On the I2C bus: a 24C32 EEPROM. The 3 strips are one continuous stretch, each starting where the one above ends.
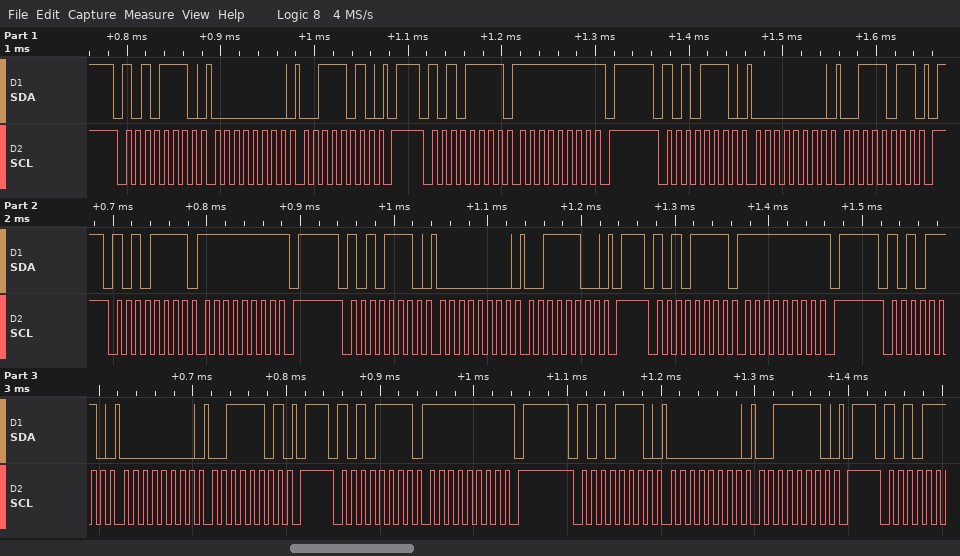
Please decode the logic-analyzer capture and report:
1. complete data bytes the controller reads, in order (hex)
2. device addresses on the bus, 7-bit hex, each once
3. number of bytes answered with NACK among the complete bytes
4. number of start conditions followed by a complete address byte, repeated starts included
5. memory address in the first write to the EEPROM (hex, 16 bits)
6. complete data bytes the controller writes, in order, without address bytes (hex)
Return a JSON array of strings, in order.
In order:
["FF FF FF FF", "0x57", "4", "9", "0x003A", "00 3A 00 3B 00 3C 00 3D 00 3E"]
